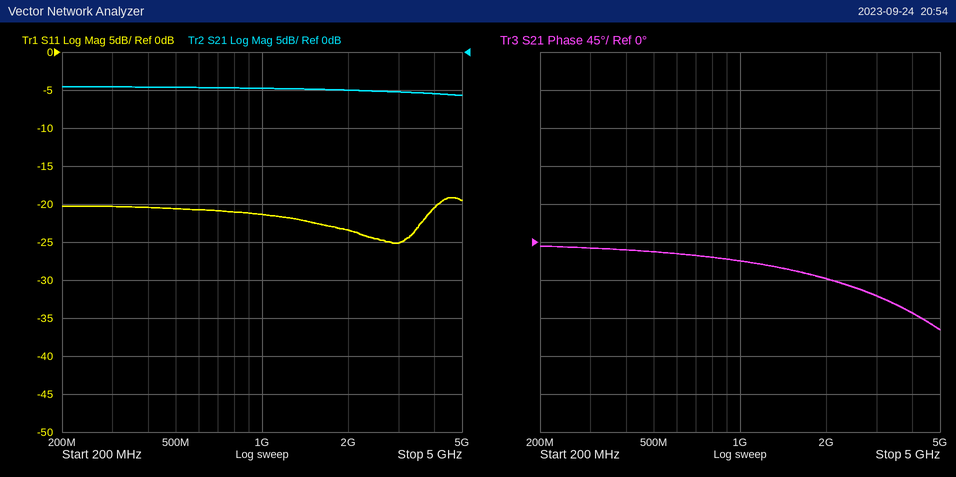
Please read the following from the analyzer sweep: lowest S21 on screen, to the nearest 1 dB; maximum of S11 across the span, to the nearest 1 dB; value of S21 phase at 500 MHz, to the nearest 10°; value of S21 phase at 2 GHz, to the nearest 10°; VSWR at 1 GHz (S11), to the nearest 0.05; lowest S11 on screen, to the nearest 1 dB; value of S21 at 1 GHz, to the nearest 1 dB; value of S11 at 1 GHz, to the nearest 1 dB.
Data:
-6 dB
-19 dB
-10°
-40°
1.20
-25 dB
-5 dB
-21 dB
